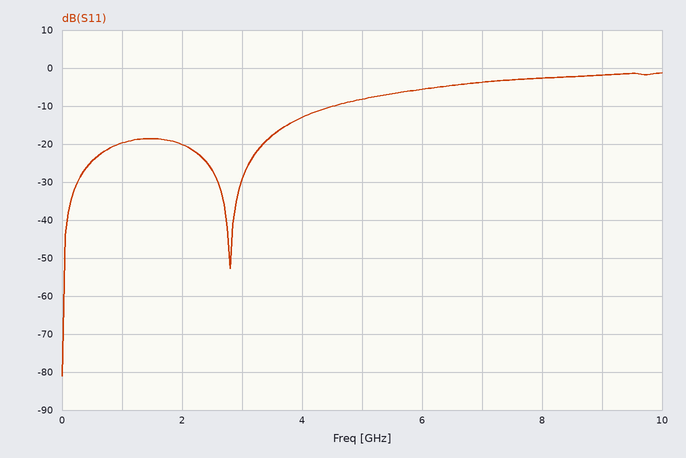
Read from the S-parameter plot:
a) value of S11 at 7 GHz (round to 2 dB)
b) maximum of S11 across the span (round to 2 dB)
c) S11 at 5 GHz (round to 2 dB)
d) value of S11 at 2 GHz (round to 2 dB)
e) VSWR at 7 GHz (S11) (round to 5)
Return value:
-4 dB
-2 dB
-8 dB
-20 dB
5
